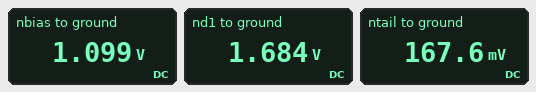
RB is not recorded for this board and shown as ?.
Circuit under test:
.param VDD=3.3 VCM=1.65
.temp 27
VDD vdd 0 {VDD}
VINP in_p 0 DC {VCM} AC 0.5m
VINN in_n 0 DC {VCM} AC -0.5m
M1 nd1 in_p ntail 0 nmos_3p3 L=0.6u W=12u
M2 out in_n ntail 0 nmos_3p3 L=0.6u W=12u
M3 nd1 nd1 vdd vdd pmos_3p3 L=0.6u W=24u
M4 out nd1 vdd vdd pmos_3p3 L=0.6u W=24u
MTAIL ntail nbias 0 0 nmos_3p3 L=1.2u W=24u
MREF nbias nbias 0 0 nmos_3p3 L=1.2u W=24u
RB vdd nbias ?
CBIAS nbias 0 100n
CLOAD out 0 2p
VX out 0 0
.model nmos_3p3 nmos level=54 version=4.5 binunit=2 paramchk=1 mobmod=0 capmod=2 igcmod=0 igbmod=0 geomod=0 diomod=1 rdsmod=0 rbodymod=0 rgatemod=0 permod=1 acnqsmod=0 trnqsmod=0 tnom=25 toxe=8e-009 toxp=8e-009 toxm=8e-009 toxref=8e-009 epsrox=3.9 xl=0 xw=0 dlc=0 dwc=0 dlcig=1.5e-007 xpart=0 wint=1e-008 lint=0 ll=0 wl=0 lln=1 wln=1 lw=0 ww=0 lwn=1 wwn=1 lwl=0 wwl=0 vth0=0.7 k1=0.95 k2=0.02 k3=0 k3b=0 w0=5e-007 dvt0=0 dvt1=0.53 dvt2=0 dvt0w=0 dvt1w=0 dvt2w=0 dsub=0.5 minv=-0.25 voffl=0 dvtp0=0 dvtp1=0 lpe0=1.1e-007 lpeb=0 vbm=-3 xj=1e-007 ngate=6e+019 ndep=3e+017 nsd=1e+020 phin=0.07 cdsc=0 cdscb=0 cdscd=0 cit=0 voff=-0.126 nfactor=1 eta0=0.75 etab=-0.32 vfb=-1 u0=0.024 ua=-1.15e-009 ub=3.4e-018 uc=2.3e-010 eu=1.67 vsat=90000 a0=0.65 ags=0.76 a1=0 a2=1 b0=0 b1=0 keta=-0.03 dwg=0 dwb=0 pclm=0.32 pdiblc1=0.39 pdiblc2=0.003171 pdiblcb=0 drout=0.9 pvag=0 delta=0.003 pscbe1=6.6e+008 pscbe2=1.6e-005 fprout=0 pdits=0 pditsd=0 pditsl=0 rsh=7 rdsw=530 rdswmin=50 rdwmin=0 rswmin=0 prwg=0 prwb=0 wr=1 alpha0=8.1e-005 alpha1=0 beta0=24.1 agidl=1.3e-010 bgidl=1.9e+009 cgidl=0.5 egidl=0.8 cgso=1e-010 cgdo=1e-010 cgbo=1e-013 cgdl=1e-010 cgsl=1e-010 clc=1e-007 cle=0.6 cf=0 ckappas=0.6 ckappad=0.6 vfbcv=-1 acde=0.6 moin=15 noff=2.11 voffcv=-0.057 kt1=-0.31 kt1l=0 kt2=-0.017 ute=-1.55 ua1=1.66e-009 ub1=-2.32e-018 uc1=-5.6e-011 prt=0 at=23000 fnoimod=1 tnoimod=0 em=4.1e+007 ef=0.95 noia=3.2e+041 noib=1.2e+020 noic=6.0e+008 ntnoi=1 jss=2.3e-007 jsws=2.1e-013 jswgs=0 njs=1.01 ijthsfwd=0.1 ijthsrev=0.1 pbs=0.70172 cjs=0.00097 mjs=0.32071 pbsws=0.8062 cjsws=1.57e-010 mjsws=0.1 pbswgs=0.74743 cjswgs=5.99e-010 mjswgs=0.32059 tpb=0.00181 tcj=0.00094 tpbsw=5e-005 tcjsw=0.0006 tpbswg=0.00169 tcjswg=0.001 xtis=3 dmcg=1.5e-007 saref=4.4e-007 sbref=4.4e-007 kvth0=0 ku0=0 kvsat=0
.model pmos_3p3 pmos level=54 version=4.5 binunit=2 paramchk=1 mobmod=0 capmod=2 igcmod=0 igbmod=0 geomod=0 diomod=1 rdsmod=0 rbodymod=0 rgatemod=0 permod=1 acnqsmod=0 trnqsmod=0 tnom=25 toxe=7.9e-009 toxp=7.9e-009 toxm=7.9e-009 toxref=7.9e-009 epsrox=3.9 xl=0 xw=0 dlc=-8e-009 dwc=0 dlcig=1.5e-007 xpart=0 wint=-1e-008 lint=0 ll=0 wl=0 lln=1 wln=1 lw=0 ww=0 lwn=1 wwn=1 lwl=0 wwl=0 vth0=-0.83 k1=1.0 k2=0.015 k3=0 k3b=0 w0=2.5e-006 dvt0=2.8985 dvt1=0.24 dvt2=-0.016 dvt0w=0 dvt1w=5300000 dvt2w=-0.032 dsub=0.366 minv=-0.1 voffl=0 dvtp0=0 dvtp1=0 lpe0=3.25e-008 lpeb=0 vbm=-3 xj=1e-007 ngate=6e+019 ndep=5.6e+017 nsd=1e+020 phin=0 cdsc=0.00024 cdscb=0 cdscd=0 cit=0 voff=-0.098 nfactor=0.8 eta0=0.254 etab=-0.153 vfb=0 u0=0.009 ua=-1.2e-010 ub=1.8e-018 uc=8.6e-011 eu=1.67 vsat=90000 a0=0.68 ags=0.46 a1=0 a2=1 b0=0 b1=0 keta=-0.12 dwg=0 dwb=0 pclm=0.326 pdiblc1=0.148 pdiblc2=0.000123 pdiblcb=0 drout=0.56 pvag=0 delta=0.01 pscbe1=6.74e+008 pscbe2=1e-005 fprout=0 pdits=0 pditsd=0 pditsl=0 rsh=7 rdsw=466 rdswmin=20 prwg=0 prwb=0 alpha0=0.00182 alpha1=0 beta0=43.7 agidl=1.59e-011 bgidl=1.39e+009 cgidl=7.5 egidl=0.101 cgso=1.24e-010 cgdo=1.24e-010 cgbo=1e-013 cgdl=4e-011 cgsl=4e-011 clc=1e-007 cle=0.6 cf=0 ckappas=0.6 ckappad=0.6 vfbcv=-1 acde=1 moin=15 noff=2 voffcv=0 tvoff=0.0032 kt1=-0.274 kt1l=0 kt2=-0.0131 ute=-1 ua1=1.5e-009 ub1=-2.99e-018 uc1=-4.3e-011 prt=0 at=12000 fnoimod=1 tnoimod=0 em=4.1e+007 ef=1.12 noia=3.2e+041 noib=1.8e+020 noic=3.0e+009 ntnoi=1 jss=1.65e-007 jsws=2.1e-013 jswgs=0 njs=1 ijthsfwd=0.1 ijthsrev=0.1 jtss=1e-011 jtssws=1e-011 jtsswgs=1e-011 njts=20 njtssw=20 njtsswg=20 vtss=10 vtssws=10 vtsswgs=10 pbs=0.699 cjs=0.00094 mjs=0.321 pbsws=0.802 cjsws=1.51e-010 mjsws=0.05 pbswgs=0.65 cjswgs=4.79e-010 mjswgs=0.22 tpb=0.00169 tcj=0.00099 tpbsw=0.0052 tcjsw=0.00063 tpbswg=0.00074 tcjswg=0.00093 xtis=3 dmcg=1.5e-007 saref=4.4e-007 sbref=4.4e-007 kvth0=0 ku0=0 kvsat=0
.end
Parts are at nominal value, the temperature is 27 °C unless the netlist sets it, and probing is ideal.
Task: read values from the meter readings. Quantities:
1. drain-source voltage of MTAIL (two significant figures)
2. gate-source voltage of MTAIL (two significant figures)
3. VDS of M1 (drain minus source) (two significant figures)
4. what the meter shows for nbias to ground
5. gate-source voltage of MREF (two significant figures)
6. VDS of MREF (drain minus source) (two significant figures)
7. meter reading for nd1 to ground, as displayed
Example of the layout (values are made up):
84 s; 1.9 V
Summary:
170 mV; 1.1 V; 1.5 V; 1.099 V; 1.1 V; 1.1 V; 1.684 V
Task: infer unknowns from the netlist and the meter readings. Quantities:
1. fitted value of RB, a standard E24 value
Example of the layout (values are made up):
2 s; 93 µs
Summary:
18 kΩ
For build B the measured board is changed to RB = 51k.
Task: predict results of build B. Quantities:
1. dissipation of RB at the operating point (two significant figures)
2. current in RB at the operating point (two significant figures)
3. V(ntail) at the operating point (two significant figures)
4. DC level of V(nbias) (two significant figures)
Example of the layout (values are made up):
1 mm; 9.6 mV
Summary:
110 µW; 46 µA; 190 mV; 950 mV
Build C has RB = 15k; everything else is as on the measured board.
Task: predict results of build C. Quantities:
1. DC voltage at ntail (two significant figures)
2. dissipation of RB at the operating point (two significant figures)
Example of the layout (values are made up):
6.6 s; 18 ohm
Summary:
160 mV; 310 µW
